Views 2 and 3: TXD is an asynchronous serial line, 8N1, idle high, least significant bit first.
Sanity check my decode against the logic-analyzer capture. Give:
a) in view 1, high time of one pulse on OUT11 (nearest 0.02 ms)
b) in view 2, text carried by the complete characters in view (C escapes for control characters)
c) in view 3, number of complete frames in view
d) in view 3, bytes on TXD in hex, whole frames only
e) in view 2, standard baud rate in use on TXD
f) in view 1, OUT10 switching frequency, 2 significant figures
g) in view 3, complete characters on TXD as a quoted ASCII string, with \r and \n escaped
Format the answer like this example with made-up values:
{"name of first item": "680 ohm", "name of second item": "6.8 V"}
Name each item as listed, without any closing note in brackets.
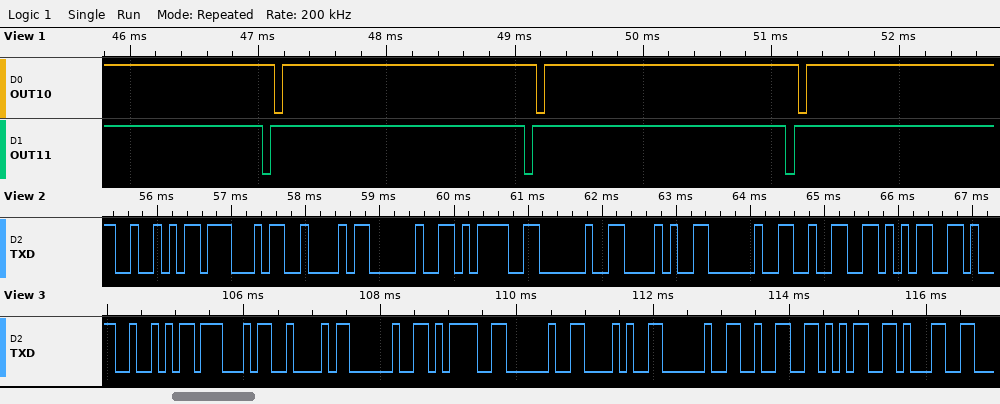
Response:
{"in view 1, high time of one pulse on OUT11": "1.98 ms", "in view 2, text carried by the complete characters in view": "\"RGB = ( 25\"", "in view 3, number of complete frames in view": "11", "in view 3, bytes on TXD in hex, whole frames only": "52 47 42 20 3D 20 28 20 32 35 31", "in view 2, standard baud rate in use on TXD": "9600 baud", "in view 1, OUT10 switching frequency, 2 significant figures": "490 Hz", "in view 3, complete characters on TXD as a quoted ASCII string, with \\r and \\n escaped": "\"RGB = ( 251\""}
